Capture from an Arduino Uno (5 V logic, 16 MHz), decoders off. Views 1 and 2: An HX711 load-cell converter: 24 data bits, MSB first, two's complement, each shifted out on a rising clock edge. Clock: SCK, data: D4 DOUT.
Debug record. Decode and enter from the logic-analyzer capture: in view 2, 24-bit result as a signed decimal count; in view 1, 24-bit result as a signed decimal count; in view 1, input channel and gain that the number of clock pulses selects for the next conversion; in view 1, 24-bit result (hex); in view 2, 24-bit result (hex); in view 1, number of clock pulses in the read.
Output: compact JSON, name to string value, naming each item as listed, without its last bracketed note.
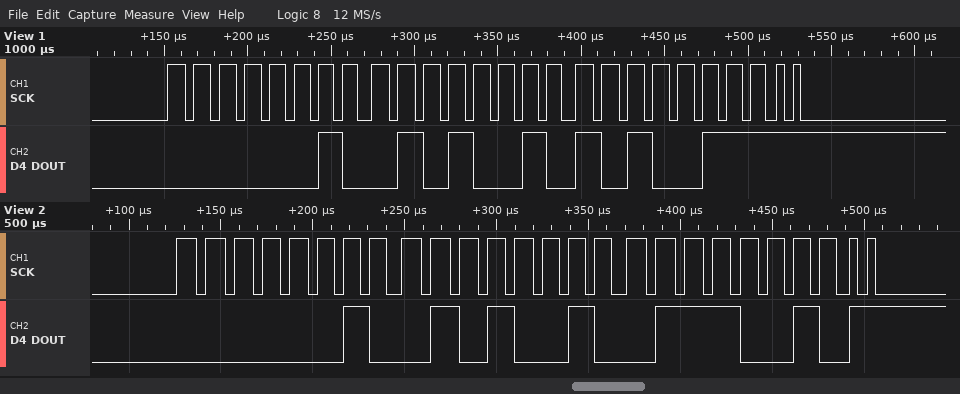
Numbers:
{"in view 2, 24-bit result as a signed decimal count": "152178", "in view 1, 24-bit result as a signed decimal count": "152231", "in view 1, input channel and gain that the number of clock pulses selects for the next conversion": "channel B, gain 32", "in view 1, 24-bit result": "0x0252A7", "in view 2, 24-bit result": "0x025272", "in view 1, number of clock pulses in the read": "26"}
